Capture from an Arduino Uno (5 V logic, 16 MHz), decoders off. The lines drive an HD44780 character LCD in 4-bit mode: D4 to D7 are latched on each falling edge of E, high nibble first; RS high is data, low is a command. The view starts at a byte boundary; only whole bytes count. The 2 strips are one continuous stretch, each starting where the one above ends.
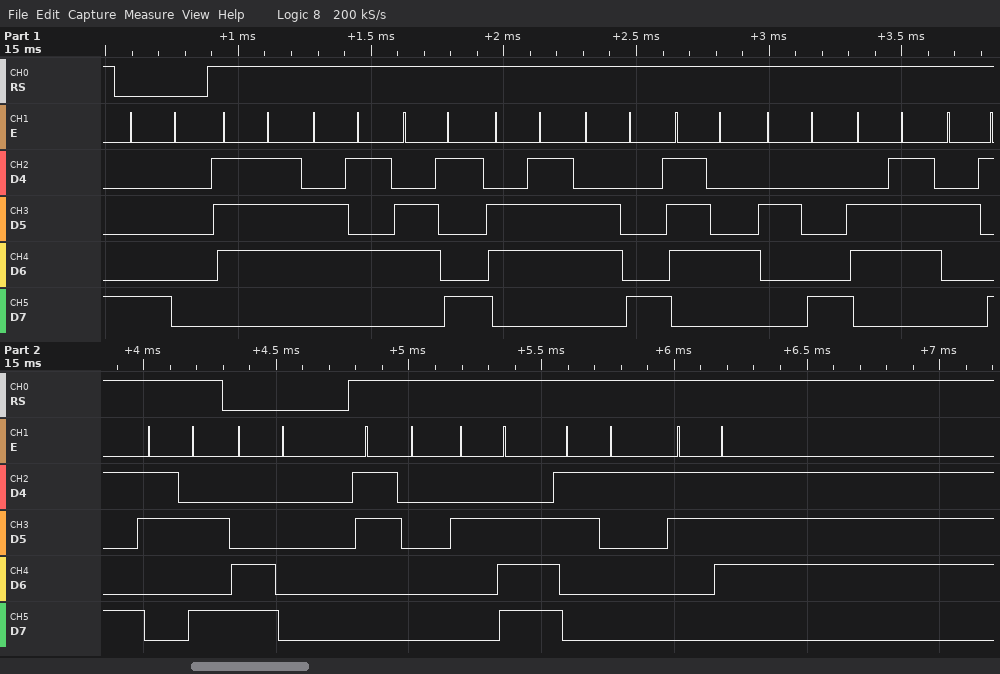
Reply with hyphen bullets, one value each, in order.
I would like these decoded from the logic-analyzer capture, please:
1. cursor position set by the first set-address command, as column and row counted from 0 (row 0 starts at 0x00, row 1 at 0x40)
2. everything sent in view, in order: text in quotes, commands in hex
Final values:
- column 0, row 0
- 0x80 "weight(g):" 0xC0 "0.17"
